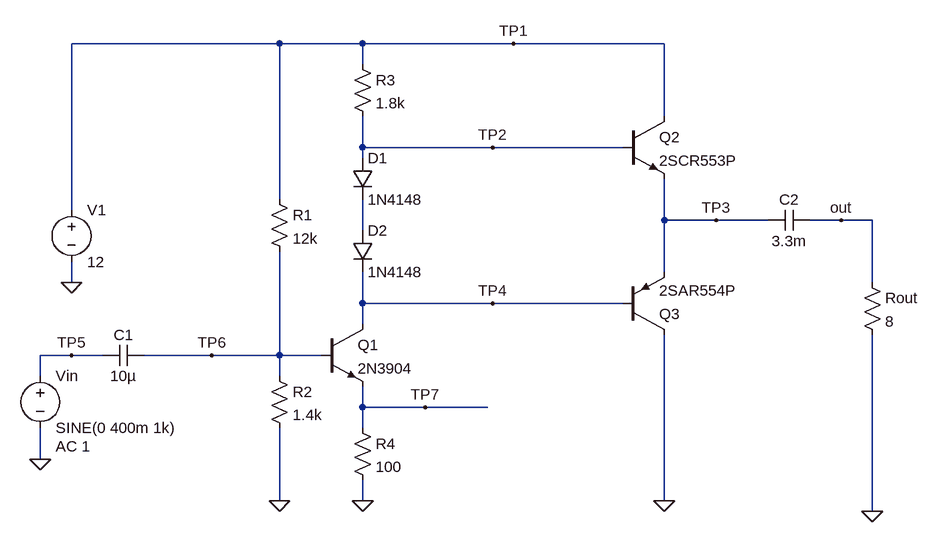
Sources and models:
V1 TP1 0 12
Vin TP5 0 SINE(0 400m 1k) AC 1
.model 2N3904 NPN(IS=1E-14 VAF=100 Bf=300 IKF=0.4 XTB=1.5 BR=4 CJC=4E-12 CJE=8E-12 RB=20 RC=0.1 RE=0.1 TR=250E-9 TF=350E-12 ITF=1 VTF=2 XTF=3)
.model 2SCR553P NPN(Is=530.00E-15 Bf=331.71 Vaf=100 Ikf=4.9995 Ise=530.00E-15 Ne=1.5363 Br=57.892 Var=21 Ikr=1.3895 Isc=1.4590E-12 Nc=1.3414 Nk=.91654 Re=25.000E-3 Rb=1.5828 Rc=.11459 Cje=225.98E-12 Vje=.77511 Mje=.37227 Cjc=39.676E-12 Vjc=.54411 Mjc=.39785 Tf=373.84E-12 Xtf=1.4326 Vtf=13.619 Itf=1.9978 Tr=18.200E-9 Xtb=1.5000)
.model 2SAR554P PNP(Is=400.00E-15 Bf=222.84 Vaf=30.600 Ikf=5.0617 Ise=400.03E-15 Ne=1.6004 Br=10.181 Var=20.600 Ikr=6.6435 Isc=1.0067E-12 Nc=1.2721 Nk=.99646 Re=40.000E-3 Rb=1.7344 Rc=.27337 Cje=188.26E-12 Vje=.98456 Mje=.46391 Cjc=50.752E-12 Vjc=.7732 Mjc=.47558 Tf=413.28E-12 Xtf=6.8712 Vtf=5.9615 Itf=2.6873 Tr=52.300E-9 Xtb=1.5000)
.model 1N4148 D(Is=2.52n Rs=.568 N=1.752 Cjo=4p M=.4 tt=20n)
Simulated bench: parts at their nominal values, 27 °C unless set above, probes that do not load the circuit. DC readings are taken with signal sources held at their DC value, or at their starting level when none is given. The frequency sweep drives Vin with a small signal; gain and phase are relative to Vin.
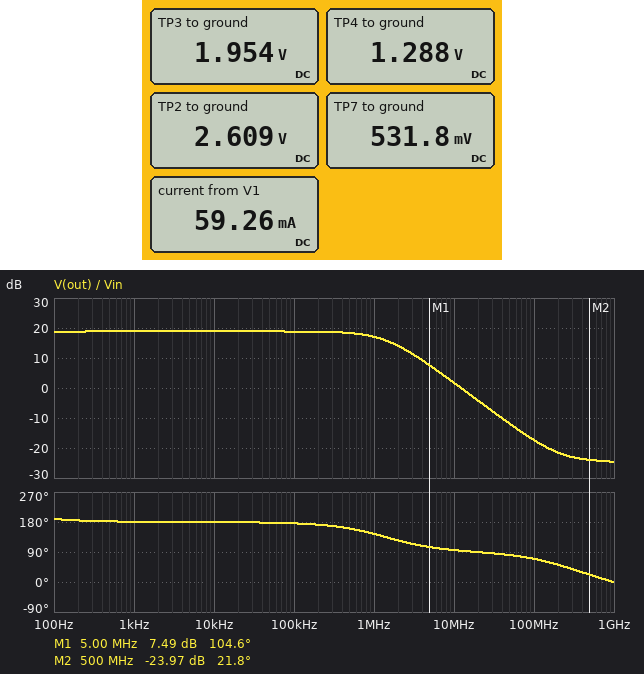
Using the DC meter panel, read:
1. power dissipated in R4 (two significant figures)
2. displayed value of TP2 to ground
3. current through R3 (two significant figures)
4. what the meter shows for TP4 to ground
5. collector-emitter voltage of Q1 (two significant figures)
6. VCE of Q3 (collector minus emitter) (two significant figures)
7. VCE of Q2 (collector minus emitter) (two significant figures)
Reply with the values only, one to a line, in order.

2.8 mW
2.609 V
5.2 mA
1.288 V
760 mV
-2.0 V
10 V
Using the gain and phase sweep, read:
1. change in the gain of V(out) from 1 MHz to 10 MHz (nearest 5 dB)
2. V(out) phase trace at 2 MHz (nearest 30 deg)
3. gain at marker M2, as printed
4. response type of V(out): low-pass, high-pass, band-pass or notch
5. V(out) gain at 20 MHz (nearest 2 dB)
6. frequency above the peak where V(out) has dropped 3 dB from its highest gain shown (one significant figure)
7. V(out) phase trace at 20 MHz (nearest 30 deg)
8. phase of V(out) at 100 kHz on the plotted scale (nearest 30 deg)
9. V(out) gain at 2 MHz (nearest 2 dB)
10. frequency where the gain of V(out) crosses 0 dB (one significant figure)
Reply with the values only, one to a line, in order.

-15 dB
120 deg
-23.97 dB
low-pass
-4 dB
1 MHz
90 deg
180 deg
14 dB
10 MHz
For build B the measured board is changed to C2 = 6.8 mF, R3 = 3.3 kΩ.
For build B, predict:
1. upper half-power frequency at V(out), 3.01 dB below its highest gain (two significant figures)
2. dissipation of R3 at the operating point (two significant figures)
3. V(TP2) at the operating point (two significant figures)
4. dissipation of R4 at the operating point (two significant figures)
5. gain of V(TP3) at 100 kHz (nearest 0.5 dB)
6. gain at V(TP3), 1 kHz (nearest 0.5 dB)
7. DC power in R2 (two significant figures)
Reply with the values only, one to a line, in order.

56 MHz
32 mW
1.7 V
1.1 mW
-9.0 dB
-18.0 dB
760 µW
